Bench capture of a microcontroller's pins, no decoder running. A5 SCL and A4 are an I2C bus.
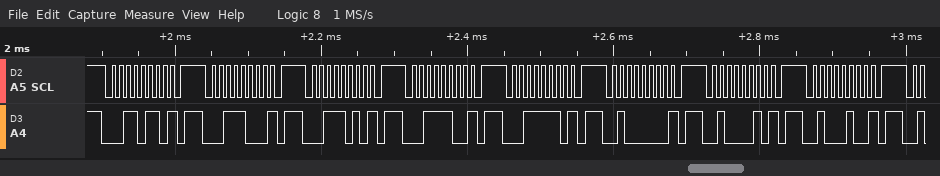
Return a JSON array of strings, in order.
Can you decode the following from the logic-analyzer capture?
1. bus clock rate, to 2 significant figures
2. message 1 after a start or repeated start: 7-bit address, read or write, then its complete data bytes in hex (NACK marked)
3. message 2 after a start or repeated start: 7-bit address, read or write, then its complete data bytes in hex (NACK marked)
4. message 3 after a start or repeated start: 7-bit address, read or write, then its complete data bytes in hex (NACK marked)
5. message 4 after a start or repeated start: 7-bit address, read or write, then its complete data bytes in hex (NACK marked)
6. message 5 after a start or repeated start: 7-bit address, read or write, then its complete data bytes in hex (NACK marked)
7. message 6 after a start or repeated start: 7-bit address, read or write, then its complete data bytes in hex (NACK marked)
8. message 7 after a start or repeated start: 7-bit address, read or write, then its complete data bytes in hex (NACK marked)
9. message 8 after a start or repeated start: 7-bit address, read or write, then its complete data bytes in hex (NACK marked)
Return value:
["100 kHz", "0x1B write NACK", "0x1C write NACK", "0x1D write NACK", "0x1E write NACK", "0x1F write NACK", "0x20 write NACK", "0x21 write NACK", "0x22 write NACK"]
